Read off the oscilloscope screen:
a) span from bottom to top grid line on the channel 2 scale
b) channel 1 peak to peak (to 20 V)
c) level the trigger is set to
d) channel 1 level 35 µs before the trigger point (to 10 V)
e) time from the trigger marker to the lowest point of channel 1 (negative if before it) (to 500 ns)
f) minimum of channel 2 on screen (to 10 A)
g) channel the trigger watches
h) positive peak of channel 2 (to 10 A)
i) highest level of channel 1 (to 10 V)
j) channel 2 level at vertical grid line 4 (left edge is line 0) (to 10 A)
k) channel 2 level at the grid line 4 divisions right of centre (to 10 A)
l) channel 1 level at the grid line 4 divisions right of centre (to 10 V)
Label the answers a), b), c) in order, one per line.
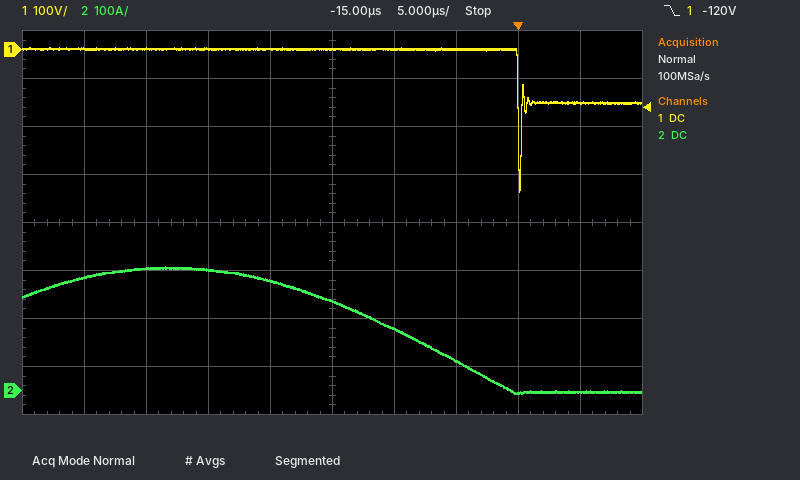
a) 800 A
b) 300 V
c) -120 V
d) 0 V
e) 0.0 µs
f) -10 A
g) channel 1
h) 260 A
i) 0 V
j) 230 A
k) 0 A
l) -110 V
